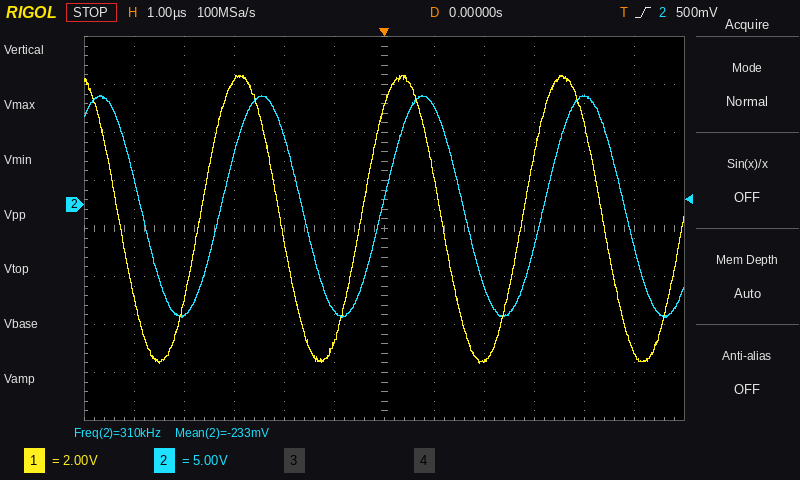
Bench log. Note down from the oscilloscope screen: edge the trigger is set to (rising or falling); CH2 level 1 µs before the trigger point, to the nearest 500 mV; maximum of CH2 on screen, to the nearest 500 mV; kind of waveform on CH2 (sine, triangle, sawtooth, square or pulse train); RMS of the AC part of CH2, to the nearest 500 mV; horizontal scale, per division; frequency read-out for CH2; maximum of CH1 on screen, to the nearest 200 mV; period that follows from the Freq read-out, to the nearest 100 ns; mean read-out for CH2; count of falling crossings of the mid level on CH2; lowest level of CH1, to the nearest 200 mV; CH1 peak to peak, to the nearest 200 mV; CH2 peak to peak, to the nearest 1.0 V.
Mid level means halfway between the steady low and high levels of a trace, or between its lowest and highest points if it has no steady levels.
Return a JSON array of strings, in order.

["rising", "-11.0 V", "11.5 V", "sine", "8.0 V", "1 µs", "310 kHz", "5.4 V", "3.2 µs", "-233 mV", "4", "-6.6 V", "12.0 V", "23.0 V"]
